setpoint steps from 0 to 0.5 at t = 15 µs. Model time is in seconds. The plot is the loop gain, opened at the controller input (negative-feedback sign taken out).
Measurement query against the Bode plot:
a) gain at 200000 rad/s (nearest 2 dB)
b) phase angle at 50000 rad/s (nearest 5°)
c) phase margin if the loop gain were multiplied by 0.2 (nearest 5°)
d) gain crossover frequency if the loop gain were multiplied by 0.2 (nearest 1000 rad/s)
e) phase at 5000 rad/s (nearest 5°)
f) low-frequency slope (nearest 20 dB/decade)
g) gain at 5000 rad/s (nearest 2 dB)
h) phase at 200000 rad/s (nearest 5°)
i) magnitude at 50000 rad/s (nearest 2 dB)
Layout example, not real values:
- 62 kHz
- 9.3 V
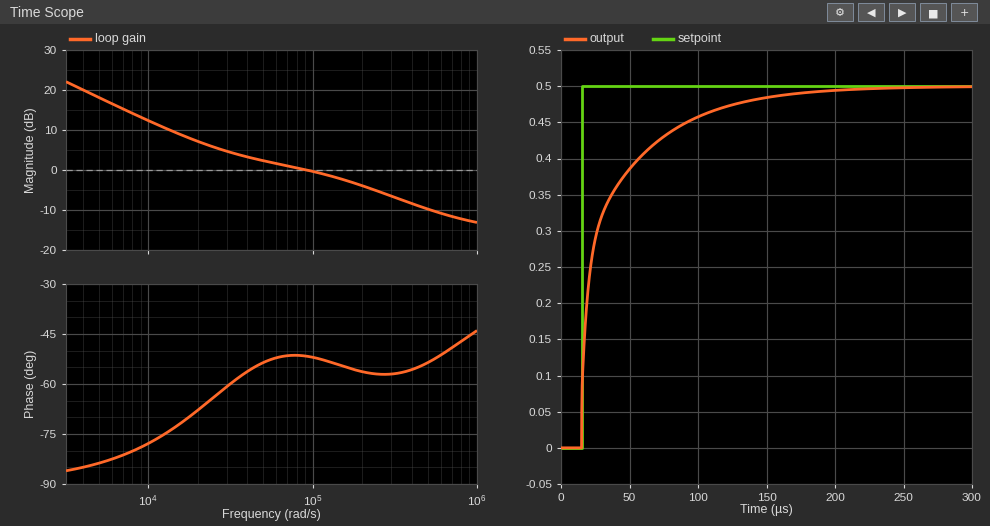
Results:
- -4 dB
- -55°
- 100°
- 8000 rad/s
- -85°
- -20 dB/decade
- 18 dB
- -55°
- 2 dB
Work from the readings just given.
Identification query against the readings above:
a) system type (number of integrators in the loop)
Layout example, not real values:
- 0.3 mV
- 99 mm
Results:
- 1
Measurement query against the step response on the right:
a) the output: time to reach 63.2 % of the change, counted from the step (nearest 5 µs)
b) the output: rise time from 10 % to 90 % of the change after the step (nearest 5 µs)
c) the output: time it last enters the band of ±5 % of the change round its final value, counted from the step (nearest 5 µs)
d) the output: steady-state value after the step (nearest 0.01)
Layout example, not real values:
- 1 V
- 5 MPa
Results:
- 15 µs
- 75 µs
- 110 µs
- 0.50
